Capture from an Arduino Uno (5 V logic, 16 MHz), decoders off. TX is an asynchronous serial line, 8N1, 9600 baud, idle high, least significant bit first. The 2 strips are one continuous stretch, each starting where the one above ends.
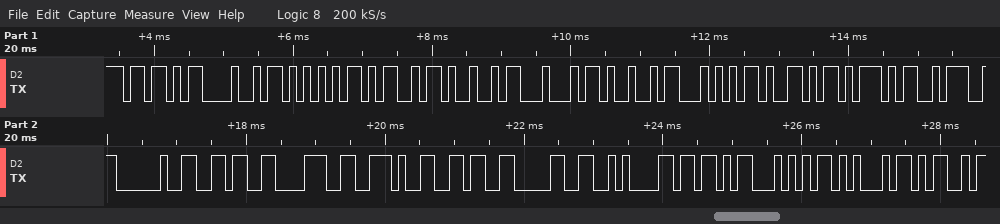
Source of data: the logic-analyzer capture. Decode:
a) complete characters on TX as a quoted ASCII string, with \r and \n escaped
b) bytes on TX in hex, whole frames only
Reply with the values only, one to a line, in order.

"[HUMIDITY]: 68.60\n[TEM"
5B 48 55 4D 49 44 49 54 59 5D 3A 20 36 38 2E 36 30 0A 5B 54 45 4D
